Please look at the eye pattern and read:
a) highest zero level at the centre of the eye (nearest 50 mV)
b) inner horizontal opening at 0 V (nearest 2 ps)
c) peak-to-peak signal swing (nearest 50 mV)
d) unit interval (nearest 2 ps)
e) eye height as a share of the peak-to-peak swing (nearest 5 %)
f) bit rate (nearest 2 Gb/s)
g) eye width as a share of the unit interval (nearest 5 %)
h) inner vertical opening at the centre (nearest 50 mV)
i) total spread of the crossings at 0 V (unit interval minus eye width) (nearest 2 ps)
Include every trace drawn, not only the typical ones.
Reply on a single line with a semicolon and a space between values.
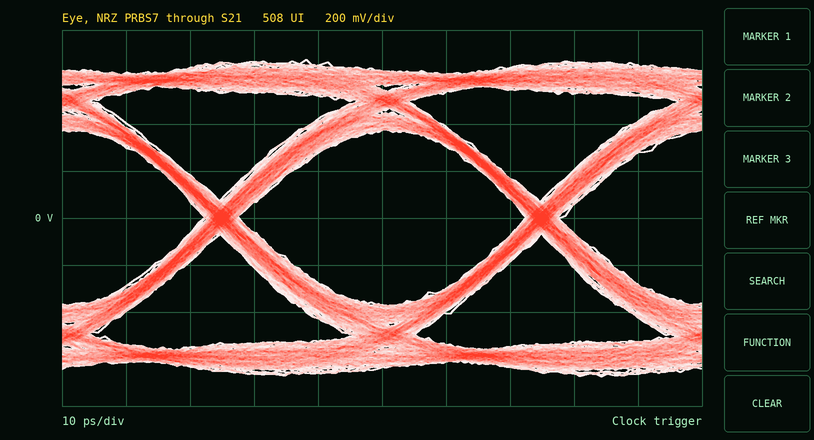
-350 mV; 44 ps; 1.35 V; 50 ps; 55 %; 20 Gb/s; 90 %; 750 mV; 6 ps
